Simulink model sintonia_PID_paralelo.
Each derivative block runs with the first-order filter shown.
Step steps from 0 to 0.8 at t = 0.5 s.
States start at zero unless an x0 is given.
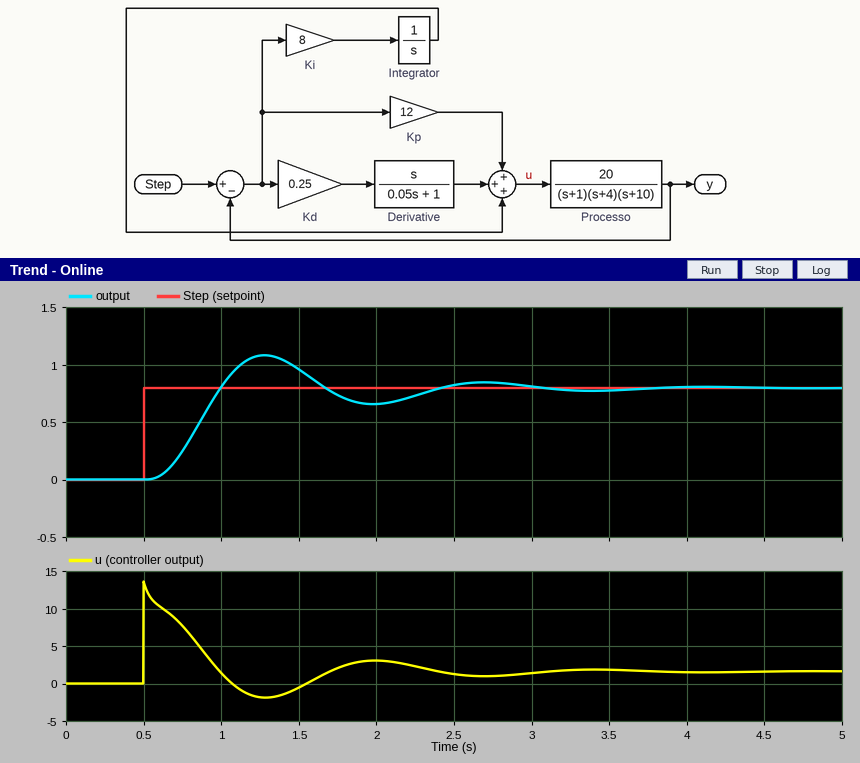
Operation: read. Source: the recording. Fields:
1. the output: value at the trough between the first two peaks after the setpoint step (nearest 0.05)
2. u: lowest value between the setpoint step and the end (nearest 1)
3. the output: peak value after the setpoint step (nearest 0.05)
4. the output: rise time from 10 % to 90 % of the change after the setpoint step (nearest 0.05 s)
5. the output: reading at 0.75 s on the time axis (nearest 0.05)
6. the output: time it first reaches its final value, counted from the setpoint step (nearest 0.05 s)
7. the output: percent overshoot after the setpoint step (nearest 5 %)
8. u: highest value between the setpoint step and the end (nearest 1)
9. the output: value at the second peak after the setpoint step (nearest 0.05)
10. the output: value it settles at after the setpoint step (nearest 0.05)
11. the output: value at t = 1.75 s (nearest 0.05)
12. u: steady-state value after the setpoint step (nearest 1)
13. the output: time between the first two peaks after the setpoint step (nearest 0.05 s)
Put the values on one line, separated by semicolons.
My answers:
0.65; -2; 1.10; 0.30 s; 0.25; 0.50 s; 35 %; 14; 0.85; 0.80; 0.75; 2; 1.40 s
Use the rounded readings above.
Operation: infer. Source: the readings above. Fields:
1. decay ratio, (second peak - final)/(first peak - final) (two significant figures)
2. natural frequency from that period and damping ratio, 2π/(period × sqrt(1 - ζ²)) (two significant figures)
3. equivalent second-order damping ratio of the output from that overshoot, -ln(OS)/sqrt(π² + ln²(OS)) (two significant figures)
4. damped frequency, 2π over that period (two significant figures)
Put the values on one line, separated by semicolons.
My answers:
0.17; 4.7 rad/s; 0.32; 4.5 rad/s
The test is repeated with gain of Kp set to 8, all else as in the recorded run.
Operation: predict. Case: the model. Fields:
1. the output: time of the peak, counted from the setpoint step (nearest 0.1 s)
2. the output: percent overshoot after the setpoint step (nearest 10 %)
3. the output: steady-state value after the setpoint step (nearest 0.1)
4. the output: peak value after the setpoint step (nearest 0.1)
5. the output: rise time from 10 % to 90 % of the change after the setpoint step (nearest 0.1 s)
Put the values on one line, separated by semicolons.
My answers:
1.0 s; 30 %; 0.8; 1.0; 0.4 s
